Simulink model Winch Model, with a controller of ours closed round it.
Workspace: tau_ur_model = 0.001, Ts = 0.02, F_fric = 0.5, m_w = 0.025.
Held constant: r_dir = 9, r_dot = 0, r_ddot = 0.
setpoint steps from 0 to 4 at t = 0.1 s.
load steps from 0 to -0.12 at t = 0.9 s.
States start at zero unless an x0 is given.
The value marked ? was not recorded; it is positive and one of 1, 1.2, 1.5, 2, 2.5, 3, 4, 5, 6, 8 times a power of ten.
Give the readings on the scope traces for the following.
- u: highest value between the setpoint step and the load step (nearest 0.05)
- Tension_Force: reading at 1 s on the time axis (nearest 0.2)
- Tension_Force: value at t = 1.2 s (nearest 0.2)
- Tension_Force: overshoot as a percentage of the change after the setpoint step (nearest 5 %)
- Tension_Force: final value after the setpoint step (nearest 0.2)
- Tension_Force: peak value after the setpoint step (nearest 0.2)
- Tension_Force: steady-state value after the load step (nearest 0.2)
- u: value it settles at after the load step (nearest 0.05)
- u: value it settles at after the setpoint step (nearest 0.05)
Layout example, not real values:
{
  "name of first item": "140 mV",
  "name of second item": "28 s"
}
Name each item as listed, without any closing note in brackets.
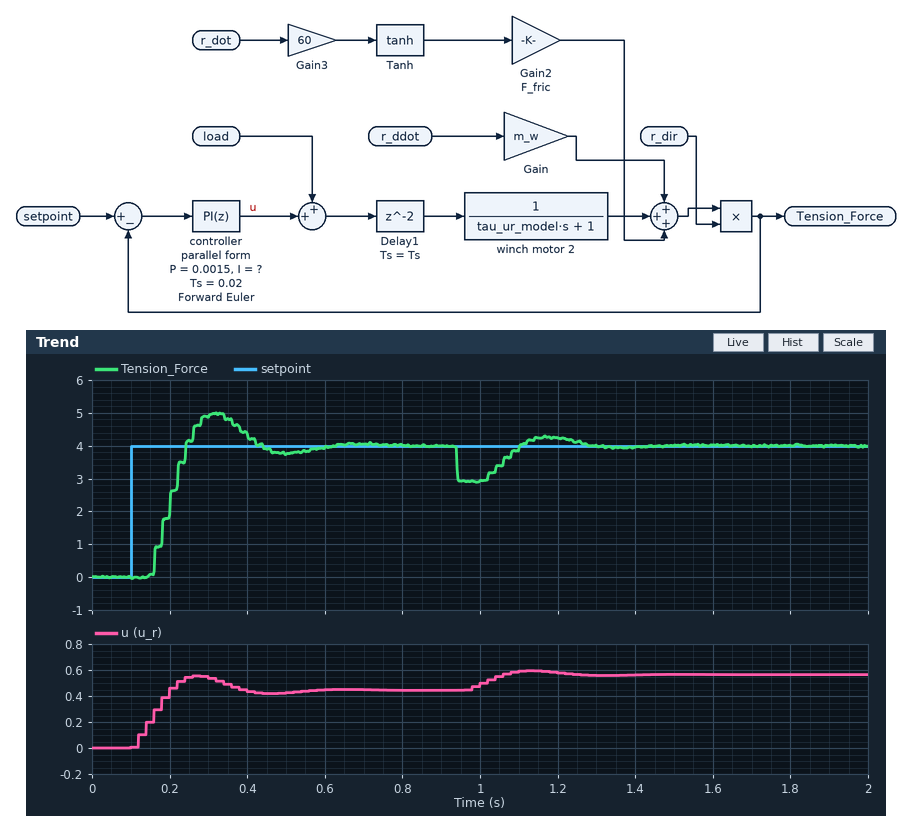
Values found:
{
  "u: highest value between the setpoint step and the load step": "0.55",
  "Tension_Force: reading at 1 s on the time axis": "3.0",
  "Tension_Force: value at t = 1.2 s": "4.2",
  "Tension_Force: overshoot as a percentage of the change after the setpoint step": "25 %",
  "Tension_Force: final value after the setpoint step": "4.0",
  "Tension_Force: peak value after the setpoint step": "5.0",
  "Tension_Force: steady-state value after the load step": "4.0",
  "u: value it settles at after the load step": "0.55",
  "u: value it settles at after the setpoint step": "0.45"
}
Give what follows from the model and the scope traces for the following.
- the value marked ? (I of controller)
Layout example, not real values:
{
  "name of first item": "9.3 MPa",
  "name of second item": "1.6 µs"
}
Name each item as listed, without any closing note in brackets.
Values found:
{
  "the value marked ?": "1.2"
}
